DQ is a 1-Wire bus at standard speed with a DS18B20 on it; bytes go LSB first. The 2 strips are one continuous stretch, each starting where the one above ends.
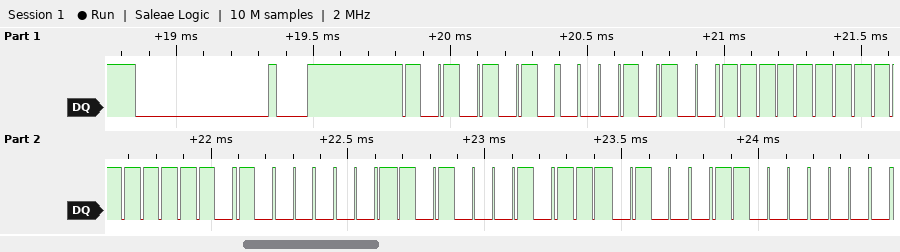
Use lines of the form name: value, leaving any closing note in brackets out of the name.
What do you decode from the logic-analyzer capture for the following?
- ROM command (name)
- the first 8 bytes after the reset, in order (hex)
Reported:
ROM command: Match ROM
the first 8 bytes after the reset, in order: 55 28 FF 7F 81 45 17 03
